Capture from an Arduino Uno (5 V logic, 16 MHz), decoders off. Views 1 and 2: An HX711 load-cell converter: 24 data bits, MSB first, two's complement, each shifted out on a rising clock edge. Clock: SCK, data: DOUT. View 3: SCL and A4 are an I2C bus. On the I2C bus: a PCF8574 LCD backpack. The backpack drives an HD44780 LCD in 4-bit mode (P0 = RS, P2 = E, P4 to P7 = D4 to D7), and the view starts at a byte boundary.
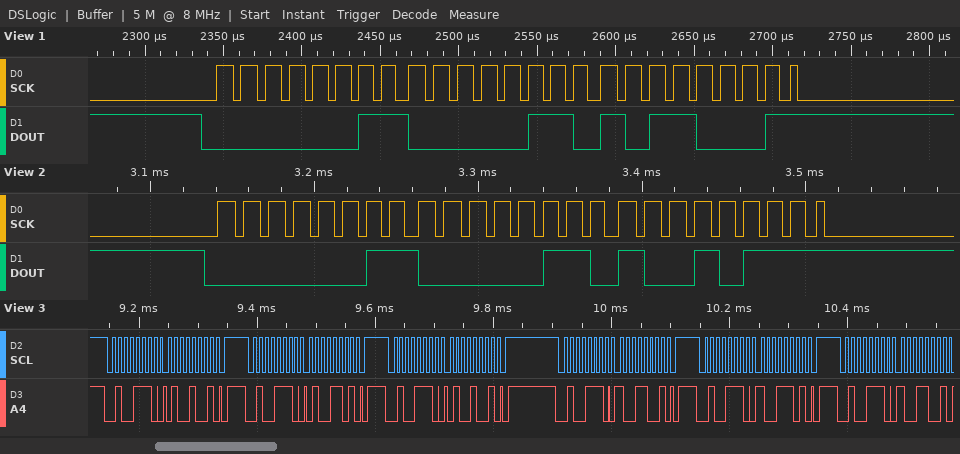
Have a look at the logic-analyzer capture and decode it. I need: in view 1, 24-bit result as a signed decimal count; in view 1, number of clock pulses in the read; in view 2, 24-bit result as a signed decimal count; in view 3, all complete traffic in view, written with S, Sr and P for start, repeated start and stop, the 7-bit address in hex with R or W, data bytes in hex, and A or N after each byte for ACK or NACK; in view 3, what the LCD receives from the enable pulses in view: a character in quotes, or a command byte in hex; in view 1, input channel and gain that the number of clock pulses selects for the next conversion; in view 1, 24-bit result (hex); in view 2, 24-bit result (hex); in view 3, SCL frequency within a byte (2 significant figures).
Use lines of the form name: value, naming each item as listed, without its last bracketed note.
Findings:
in view 1, 24-bit result as a signed decimal count: 198321
in view 1, number of clock pulses in the read: 25
in view 2, 24-bit result as a signed decimal count: 198295
in view 3, all complete traffic in view, written with S, Sr and P for start, repeated start and stop, the 7-bit address in hex with R or W, data bytes in hex, and A or N after each byte for ACK or NACK: S 27W A 49 A P S 27W A 4D A P S 27W A 49 A P S 27W A 99 A P S 27W A 9D A P S 27W A 99 A
in view 3, what the LCD receives from the enable pulses in view: a character in quotes, or a command byte in hex: 'I'
in view 1, input channel and gain that the number of clock pulses selects for the next conversion: channel A, gain 128
in view 1, 24-bit result: 0x0306B1
in view 2, 24-bit result: 0x030697
in view 3, SCL frequency within a byte: 100 kHz
